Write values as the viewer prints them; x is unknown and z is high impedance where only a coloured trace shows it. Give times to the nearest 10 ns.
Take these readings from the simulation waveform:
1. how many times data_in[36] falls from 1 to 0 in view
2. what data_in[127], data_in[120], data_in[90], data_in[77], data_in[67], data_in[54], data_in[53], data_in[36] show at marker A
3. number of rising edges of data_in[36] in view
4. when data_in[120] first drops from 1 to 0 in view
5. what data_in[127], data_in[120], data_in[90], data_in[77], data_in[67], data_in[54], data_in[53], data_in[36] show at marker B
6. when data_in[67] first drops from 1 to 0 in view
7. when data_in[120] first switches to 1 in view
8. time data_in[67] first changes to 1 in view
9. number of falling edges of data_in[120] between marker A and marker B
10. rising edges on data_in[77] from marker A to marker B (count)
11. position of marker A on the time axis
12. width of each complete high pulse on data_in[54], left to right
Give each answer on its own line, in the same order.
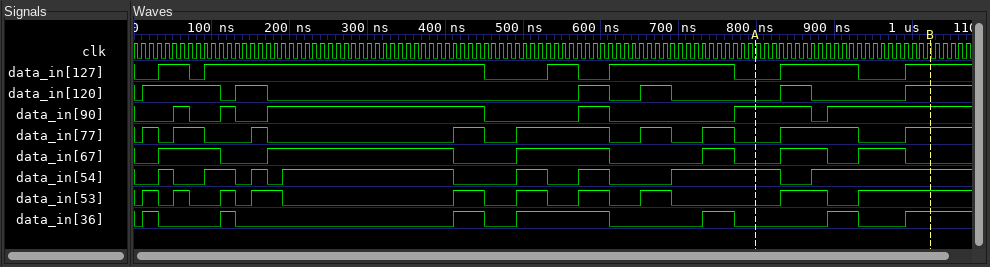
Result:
6
data_in[127]=0, data_in[120]=0, data_in[90]=1, data_in[77]=0, data_in[67]=0, data_in[54]=1, data_in[53]=0, data_in[36]=0
7
110 ns
data_in[127]=1, data_in[120]=1, data_in[90]=1, data_in[77]=1, data_in[67]=0, data_in[54]=1, data_in[53]=1, data_in[36]=1
110 ns
10 ns
30 ns
1
2
800 ns
20 ns, 40 ns, 20 ns, 220 ns, 40 ns, 40 ns, 140 ns
